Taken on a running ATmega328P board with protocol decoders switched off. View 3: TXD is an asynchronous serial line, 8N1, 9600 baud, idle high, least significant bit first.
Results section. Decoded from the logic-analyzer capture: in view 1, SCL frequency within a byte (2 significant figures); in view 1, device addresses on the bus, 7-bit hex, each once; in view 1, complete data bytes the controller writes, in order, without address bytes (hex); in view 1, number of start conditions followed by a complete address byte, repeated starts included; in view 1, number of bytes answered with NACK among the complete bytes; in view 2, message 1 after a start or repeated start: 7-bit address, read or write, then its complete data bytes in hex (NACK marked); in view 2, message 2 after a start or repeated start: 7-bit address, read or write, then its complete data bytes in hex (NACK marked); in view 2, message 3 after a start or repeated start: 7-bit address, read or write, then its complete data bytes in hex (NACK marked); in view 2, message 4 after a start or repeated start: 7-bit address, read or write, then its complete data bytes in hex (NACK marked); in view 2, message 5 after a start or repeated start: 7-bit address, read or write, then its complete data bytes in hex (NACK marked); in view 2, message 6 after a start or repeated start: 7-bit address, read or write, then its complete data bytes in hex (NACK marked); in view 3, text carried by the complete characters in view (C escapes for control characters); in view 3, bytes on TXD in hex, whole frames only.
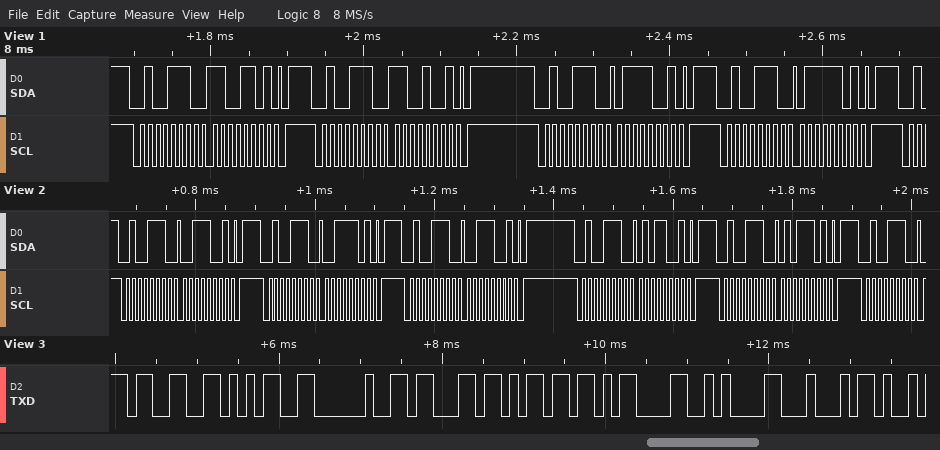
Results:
100 kHz
0x27
CD C9 79 7D
4
0
0x27 write: 39
0x27 write: 3D
0x27 write: 39
0x27 write: 59
0x27 write: 5D
0x27 write
"35 cm\r\nD"
33 35 20 63 6D 0D 0A 44
